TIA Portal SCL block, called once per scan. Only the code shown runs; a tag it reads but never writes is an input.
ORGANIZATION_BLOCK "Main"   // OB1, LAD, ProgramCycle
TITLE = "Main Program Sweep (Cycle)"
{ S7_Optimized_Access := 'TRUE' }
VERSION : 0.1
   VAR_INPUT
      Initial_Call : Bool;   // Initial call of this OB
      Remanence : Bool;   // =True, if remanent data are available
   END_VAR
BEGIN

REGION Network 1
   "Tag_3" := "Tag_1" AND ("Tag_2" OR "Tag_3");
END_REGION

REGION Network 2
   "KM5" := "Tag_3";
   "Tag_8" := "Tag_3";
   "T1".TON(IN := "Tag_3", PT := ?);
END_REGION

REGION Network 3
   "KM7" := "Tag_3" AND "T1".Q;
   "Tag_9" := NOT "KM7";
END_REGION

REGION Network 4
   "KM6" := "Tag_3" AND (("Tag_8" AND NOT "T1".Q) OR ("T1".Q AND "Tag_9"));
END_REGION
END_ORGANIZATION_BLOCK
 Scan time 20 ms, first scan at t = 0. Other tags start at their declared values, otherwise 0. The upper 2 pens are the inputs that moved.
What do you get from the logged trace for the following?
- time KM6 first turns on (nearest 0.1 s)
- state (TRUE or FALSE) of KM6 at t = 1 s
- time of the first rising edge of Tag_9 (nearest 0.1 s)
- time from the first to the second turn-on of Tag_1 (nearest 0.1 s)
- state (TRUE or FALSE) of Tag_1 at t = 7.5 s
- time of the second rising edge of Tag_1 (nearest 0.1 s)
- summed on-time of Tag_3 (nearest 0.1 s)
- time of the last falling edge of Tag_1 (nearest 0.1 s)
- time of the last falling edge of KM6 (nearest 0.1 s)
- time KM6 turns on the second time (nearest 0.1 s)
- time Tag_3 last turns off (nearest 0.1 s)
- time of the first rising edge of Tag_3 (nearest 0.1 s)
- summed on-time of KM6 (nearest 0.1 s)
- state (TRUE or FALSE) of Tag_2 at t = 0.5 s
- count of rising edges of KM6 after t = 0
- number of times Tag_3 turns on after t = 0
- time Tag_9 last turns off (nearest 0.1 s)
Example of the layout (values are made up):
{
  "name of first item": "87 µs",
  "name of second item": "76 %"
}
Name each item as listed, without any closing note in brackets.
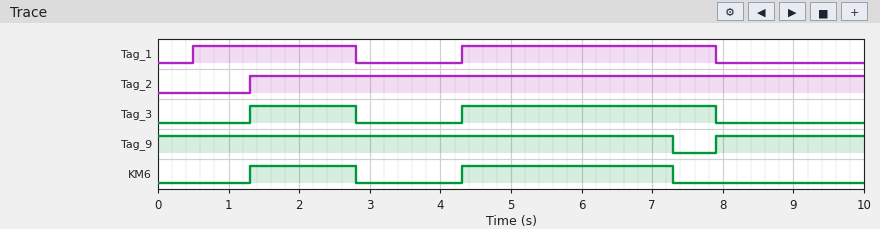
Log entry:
{
  "time KM6 first turns on": "1.3 s",
  "state (TRUE or FALSE) of KM6 at t = 1 s": "FALSE",
  "time of the first rising edge of Tag_9": "7.9 s",
  "time from the first to the second turn-on of Tag_1": "3.8 s",
  "state (TRUE or FALSE) of Tag_1 at t = 7.5 s": "TRUE",
  "time of the second rising edge of Tag_1": "4.3 s",
  "summed on-time of Tag_3": "5.1 s",
  "time of the last falling edge of Tag_1": "7.9 s",
  "time of the last falling edge of KM6": "7.3 s",
  "time KM6 turns on the second time": "4.3 s",
  "time Tag_3 last turns off": "7.9 s",
  "time of the first rising edge of Tag_3": "1.3 s",
  "summed on-time of KM6": "4.5 s",
  "state (TRUE or FALSE) of Tag_2 at t = 0.5 s": "FALSE",
  "count of rising edges of KM6 after t = 0": "2",
  "number of times Tag_3 turns on after t = 0": "2",
  "time Tag_9 last turns off": "7.3 s"
}
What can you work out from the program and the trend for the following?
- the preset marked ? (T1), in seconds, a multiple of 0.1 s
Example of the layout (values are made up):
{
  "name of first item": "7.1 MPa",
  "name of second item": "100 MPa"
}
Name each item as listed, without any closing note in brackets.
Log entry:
{
  "the preset marked ? (T1), in seconds, a multiple of 0.1 s": "3.0 s"
}
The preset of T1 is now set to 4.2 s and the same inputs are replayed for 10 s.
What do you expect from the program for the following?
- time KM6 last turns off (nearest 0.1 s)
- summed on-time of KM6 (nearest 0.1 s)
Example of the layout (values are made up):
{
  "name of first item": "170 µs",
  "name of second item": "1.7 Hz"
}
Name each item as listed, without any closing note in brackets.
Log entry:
{
  "time KM6 last turns off": "7.9 s",
  "summed on-time of KM6": "5.1 s"
}
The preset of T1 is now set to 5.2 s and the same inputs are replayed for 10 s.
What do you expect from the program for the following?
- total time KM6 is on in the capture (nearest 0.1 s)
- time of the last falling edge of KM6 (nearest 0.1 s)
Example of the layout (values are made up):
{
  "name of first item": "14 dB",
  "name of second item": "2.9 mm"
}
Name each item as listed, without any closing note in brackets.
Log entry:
{
  "total time KM6 is on in the capture": "5.1 s",
  "time of the last falling edge of KM6": "7.9 s"
}
